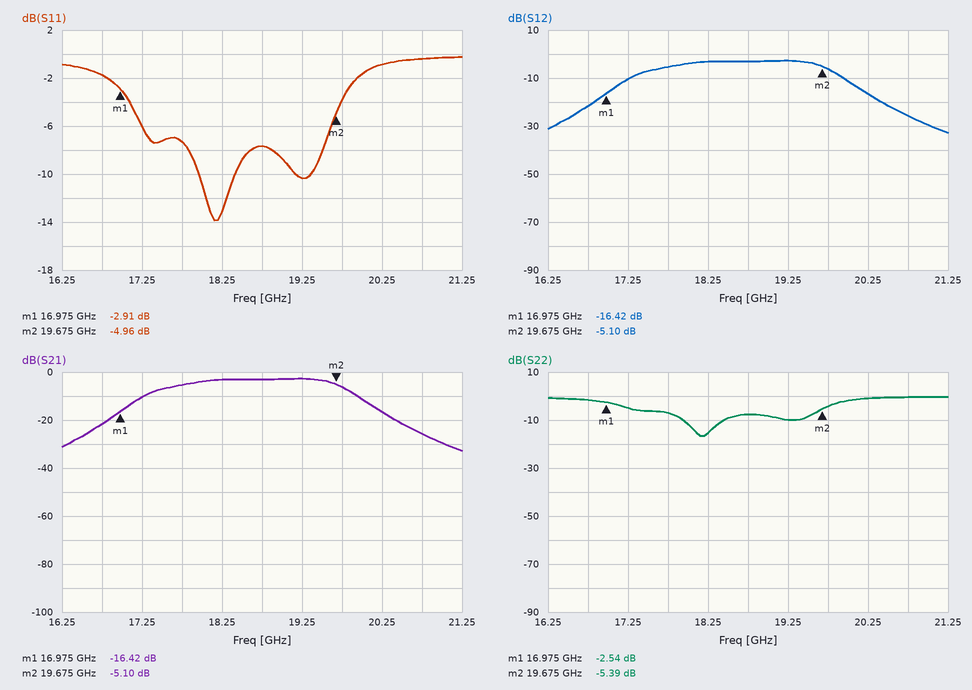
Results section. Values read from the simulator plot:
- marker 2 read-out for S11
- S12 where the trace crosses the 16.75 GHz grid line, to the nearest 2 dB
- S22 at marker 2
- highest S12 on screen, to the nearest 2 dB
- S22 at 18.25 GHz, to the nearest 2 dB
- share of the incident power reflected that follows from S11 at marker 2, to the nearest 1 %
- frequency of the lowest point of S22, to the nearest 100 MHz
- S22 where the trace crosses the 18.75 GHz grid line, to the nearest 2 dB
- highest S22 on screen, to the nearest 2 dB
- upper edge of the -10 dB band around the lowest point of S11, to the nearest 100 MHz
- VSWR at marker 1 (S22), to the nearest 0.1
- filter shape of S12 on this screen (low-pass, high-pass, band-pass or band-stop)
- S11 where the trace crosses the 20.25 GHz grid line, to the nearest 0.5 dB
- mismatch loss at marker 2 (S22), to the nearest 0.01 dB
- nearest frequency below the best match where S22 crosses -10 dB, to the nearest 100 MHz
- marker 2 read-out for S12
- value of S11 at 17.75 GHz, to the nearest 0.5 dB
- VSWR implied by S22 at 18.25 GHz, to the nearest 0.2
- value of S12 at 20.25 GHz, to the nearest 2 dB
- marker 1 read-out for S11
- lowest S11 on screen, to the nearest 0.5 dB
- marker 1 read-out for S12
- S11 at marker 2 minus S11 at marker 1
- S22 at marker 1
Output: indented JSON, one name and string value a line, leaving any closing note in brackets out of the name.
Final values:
{
  "marker 2 read-out for S11": "-4.96 dB",
  "S12 where the trace crosses the 16.75 GHz grid line, to the nearest 2 dB": "-22 dB",
  "S22 at marker 2": "-5.39 dB",
  "highest S12 on screen, to the nearest 2 dB": "-2 dB",
  "S22 at 18.25 GHz, to the nearest 2 dB": "-16 dB",
  "share of the incident power reflected that follows from S11 at marker 2, to the nearest 1 %": "32 %",
  "frequency of the lowest point of S22, to the nearest 100 MHz": "18.2 GHz",
  "S22 where the trace crosses the 18.75 GHz grid line, to the nearest 2 dB": "-8 dB",
  "highest S22 on screen, to the nearest 2 dB": "0 dB",
  "upper edge of the -10 dB band around the lowest point of S11, to the nearest 100 MHz": "18.4 GHz",
  "VSWR at marker 1 (S22), to the nearest 0.1": "6.9",
  "filter shape of S12 on this screen": "band-pass",
  "S11 where the trace crosses the 20.25 GHz grid line, to the nearest 0.5 dB": "-1.0 dB",
  "mismatch loss at marker 2 (S22), to the nearest 0.01 dB": "1.48 dB",
  "nearest frequency below the best match where S22 crosses -10 dB, to the nearest 100 MHz": "17.9 GHz",
  "marker 2 read-out for S12": "-5.10 dB",
  "value of S11 at 17.75 GHz, to the nearest 0.5 dB": "-7.5 dB",
  "VSWR implied by S22 at 18.25 GHz, to the nearest 0.2": "1.4",
  "value of S12 at 20.25 GHz, to the nearest 2 dB": "-16 dB",
  "marker 1 read-out for S11": "-2.91 dB",
  "lowest S11 on screen, to the nearest 0.5 dB": "-14.0 dB",
  "marker 1 read-out for S12": "-16.42 dB",
  "S11 at marker 2 minus S11 at marker 1": "-2.05 dB",
  "S22 at marker 1": "-2.54 dB"
}
